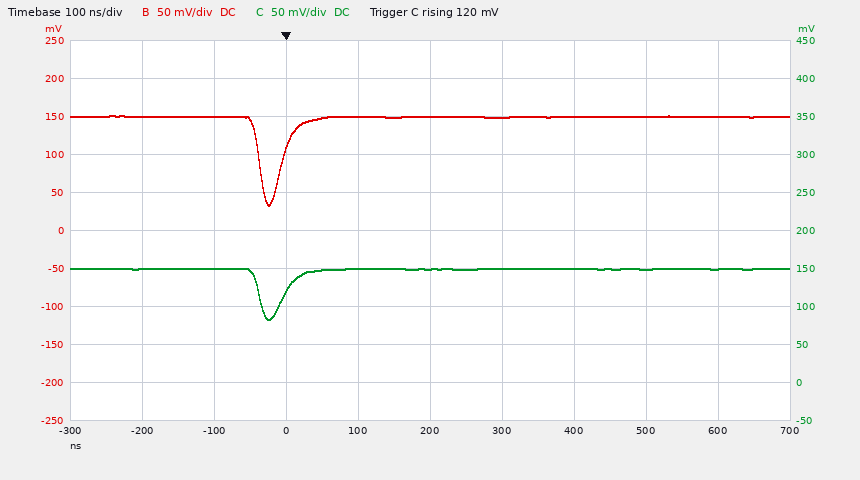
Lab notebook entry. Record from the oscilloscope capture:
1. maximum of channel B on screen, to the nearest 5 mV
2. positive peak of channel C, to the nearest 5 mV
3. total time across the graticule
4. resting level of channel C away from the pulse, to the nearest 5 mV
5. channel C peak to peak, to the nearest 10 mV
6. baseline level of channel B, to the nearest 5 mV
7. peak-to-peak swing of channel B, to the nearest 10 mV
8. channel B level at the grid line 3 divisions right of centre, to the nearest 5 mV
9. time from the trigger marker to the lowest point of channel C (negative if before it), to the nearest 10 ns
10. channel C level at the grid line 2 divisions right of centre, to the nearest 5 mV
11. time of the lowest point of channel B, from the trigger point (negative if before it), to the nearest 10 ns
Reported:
150 mV
150 mV
1 µs
150 mV
70 mV
150 mV
120 mV
150 mV
-20 ns
150 mV
-20 ns
